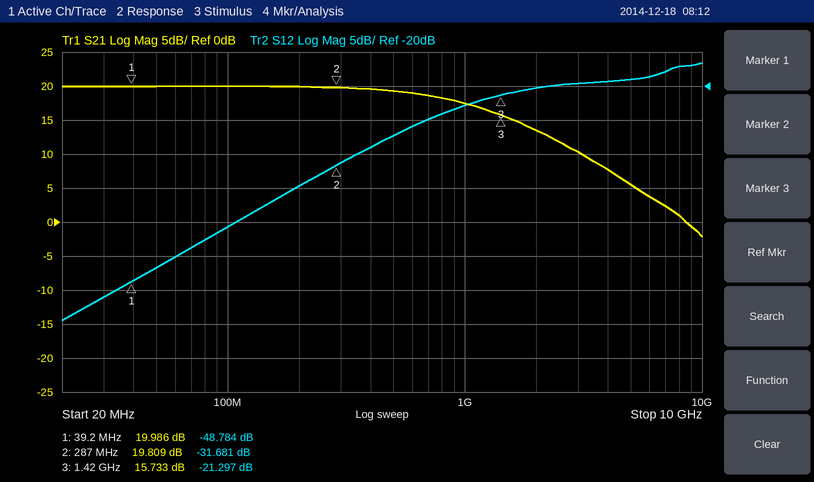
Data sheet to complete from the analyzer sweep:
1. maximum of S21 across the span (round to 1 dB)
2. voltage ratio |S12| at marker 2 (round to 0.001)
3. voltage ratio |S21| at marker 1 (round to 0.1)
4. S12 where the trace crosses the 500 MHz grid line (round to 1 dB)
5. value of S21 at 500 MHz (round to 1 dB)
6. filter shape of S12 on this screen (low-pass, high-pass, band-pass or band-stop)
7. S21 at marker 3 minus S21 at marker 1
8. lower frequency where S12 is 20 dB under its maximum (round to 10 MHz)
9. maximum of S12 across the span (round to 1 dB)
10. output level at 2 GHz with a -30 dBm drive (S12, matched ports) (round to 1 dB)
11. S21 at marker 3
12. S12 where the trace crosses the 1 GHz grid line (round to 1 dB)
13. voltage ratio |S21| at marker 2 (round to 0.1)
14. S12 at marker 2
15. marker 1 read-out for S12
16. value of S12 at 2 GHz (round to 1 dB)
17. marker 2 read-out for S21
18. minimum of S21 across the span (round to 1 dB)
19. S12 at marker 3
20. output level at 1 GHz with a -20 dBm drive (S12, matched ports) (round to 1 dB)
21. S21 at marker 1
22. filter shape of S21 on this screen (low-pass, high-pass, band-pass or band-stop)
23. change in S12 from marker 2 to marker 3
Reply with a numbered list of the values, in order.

1. 20 dB
2. 0.026
3. 10.0
4. -27 dB
5. 19 dB
6. high-pass
7. -4.253 dB
8. 160 MHz
9. -17 dB
10. -50 dBm
11. 15.733 dB
12. -23 dB
13. 9.8
14. -31.681 dB
15. -48.784 dB
16. -20 dB
17. 19.809 dB
18. -2 dB
19. -21.297 dB
20. -43 dBm
21. 19.986 dB
22. low-pass
23. 10.384 dB
